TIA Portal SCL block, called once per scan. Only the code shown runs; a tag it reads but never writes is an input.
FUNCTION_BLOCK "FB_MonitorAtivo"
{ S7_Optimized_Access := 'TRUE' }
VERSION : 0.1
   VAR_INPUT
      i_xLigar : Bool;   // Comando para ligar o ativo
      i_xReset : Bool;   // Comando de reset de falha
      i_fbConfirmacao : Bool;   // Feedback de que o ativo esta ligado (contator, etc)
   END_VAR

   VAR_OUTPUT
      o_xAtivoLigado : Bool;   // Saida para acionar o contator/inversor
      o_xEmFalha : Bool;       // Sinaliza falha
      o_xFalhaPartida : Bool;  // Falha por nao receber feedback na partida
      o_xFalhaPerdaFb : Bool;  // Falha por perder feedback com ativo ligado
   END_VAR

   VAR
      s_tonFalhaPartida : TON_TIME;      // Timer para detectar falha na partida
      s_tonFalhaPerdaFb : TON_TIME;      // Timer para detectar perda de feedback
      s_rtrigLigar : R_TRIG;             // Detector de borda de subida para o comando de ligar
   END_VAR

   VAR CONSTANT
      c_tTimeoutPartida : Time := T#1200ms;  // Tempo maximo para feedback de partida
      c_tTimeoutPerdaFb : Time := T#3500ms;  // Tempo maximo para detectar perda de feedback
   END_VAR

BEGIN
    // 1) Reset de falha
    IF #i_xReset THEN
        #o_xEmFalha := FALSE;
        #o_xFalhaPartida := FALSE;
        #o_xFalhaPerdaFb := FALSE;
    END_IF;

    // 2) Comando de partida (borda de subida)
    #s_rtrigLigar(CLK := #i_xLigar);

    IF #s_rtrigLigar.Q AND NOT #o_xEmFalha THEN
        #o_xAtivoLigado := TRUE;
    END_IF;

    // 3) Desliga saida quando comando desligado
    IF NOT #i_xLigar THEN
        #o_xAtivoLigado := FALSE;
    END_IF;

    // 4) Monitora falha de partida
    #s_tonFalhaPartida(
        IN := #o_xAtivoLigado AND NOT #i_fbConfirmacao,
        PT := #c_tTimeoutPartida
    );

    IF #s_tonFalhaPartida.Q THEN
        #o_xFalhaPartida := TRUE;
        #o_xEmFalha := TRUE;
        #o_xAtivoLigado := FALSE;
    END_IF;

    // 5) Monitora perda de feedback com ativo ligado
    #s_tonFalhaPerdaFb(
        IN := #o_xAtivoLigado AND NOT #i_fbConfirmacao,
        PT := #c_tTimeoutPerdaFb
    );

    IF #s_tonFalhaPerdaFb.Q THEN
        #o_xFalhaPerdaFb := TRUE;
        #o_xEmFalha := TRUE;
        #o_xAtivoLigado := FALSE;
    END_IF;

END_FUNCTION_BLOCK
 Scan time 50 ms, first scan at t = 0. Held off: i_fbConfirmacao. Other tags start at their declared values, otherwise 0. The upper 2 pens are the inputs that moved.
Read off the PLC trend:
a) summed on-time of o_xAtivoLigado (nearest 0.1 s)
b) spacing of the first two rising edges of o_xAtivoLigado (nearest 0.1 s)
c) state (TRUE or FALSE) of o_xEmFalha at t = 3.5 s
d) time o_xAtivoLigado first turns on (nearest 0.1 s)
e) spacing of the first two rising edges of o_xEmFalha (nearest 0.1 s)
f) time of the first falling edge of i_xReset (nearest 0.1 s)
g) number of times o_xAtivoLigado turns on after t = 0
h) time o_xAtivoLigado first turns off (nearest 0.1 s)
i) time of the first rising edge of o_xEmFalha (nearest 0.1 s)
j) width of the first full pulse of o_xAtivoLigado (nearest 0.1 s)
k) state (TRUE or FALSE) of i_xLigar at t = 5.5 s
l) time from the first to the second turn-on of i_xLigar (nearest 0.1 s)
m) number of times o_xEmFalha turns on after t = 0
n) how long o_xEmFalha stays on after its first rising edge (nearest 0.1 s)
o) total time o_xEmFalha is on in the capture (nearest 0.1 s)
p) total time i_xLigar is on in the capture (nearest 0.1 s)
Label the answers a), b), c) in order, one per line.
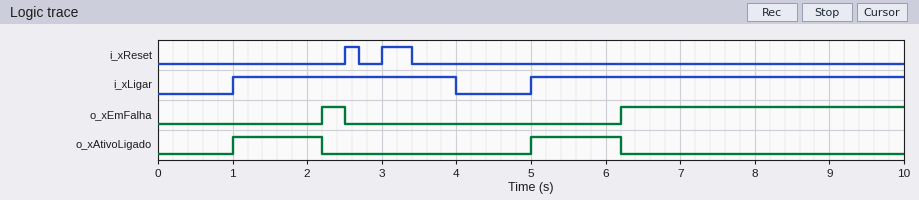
a) 2.4 s
b) 4.0 s
c) FALSE
d) 1.0 s
e) 4.0 s
f) 2.7 s
g) 2
h) 2.2 s
i) 2.2 s
j) 1.2 s
k) TRUE
l) 4.0 s
m) 2
n) 0.3 s
o) 4.1 s
p) 8.0 s
